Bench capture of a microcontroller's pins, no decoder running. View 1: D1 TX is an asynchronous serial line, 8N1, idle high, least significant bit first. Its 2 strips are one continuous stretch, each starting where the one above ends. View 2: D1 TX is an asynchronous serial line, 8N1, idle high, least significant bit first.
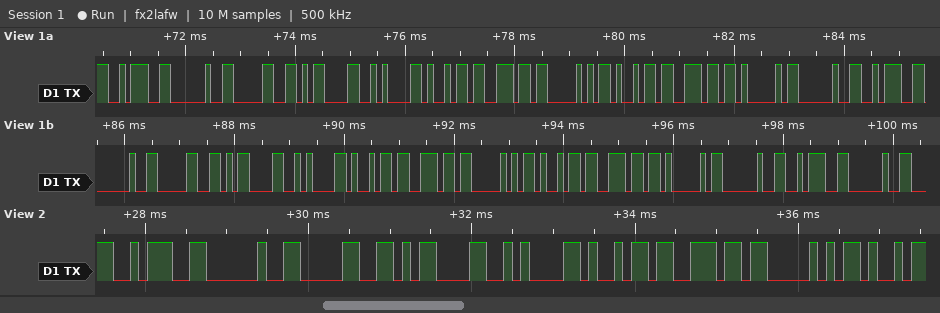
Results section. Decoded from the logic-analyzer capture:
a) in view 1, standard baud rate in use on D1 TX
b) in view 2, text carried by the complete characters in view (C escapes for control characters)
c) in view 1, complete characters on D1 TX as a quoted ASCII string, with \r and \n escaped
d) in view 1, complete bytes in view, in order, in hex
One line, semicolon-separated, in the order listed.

9600 baud; ": 0\r\ninP"; ": 0\r\ninPinA : 0\r\ninPinA : "; 3A 20 30 0D 0A 69 6E 50 69 6E 41 20 3A 20 30 0D 0A 69 6E 50 69 6E 41 20 3A 20
